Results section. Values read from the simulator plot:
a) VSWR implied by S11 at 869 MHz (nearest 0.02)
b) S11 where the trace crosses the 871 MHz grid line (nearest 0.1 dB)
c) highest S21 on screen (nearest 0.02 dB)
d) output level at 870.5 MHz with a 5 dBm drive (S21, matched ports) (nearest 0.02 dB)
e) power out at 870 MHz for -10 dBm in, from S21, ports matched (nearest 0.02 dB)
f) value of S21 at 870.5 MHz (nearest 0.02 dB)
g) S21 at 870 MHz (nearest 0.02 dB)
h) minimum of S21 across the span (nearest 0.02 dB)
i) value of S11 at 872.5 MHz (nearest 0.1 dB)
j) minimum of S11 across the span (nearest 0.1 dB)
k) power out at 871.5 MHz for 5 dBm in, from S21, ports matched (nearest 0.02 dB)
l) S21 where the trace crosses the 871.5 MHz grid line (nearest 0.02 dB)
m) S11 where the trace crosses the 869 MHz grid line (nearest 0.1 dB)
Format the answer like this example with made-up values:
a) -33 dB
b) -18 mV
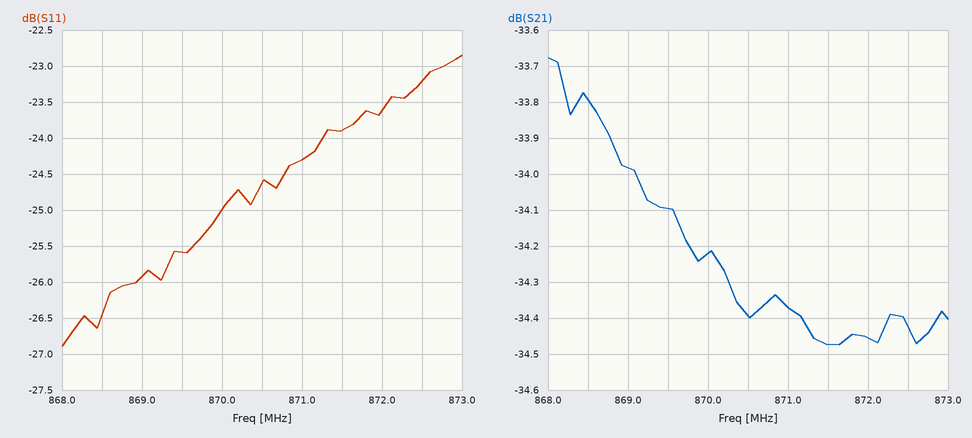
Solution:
a) 1.10
b) -24.3 dB
c) -33.68 dB
d) -29.40 dBm
e) -44.22 dBm
f) -34.40 dB
g) -34.22 dB
h) -34.48 dB
i) -23.2 dB
j) -26.9 dB
k) -29.48 dBm
l) -34.48 dB
m) -25.9 dB
